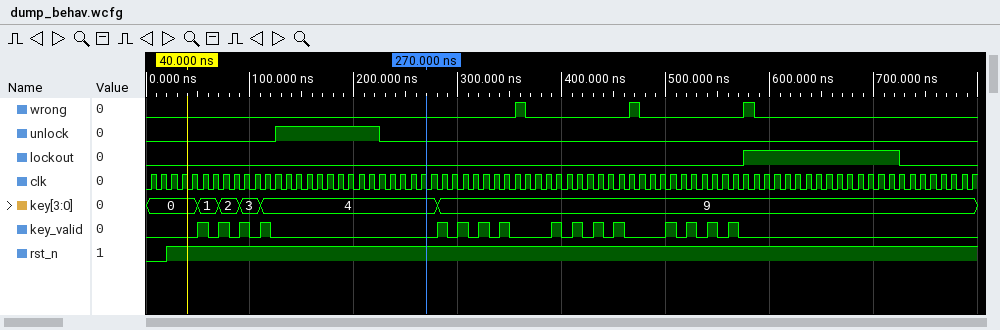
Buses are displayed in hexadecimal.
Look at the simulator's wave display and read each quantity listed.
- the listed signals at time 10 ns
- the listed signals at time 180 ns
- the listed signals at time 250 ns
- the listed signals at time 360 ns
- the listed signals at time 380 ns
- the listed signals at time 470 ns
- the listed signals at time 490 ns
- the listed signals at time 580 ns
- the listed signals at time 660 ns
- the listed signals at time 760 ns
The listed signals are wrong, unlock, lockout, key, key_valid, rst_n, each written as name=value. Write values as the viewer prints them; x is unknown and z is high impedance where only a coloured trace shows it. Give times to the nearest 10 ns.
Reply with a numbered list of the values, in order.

1. wrong=0, unlock=0, lockout=0, key=0, key_valid=0, rst_n=0
2. wrong=0, unlock=1, lockout=0, key=4, key_valid=0, rst_n=1
3. wrong=0, unlock=0, lockout=0, key=4, key_valid=0, rst_n=1
4. wrong=1, unlock=0, lockout=0, key=9, key_valid=0, rst_n=1
5. wrong=0, unlock=0, lockout=0, key=9, key_valid=0, rst_n=1
6. wrong=1, unlock=0, lockout=0, key=9, key_valid=0, rst_n=1
7. wrong=0, unlock=0, lockout=0, key=9, key_valid=0, rst_n=1
8. wrong=1, unlock=0, lockout=1, key=9, key_valid=0, rst_n=1
9. wrong=0, unlock=0, lockout=1, key=9, key_valid=0, rst_n=1
10. wrong=0, unlock=0, lockout=0, key=9, key_valid=0, rst_n=1
